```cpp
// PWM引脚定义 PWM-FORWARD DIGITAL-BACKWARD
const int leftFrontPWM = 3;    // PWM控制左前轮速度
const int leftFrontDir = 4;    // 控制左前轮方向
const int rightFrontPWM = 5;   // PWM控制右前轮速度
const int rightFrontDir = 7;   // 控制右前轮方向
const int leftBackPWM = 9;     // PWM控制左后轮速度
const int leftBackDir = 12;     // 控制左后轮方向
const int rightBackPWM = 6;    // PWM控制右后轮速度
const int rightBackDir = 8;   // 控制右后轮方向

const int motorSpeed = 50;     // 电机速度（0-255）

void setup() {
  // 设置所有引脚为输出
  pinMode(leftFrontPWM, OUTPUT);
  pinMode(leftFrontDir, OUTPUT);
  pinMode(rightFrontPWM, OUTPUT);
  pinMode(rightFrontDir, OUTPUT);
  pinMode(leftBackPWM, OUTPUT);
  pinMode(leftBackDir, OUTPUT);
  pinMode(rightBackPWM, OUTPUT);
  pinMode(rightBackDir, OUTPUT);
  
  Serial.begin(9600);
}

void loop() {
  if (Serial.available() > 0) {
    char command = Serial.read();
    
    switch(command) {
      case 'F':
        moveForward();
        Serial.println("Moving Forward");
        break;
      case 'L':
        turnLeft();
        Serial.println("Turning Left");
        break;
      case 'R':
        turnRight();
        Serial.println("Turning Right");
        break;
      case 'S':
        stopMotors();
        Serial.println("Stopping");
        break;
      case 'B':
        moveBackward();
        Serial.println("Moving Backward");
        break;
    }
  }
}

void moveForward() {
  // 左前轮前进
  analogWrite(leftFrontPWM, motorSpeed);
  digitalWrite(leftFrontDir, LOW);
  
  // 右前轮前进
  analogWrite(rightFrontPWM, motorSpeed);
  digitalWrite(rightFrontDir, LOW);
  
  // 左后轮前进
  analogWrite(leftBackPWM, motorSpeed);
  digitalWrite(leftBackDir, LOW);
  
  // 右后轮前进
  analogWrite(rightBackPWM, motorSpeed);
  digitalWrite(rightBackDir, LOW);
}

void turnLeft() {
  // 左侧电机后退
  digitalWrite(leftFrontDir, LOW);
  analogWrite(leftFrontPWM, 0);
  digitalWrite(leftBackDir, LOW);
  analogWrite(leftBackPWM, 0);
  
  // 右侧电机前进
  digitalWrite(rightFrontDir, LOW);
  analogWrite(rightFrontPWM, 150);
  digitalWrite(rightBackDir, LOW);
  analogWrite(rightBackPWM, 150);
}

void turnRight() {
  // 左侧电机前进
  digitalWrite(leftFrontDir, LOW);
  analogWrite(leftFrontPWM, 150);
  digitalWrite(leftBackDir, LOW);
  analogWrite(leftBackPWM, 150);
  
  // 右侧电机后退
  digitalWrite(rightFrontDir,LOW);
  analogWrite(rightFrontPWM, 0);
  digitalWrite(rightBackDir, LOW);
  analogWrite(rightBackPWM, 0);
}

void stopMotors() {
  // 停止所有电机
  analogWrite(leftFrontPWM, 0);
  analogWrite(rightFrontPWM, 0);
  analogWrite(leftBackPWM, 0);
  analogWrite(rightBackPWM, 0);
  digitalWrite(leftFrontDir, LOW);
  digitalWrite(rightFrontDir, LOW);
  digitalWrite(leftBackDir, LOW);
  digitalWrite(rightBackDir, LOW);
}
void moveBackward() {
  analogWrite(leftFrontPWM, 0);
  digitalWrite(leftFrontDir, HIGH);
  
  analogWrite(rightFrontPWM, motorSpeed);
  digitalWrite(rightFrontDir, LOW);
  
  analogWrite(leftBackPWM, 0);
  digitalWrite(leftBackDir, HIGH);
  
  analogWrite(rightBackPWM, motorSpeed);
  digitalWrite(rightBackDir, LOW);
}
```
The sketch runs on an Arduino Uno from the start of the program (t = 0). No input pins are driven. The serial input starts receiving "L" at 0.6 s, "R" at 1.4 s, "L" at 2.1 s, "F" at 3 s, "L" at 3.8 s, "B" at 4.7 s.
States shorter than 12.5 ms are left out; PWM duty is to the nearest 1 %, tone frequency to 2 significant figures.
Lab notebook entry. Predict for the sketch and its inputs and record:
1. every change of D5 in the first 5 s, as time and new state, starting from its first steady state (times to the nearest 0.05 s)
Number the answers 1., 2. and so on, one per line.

1. 0 s low; 0.6 s PWM 59 %; 1.4 s low; 2.1 s PWM 59 %; 3 s PWM 20 %; 3.8 s PWM 59 %; 4.7 s PWM 20 %
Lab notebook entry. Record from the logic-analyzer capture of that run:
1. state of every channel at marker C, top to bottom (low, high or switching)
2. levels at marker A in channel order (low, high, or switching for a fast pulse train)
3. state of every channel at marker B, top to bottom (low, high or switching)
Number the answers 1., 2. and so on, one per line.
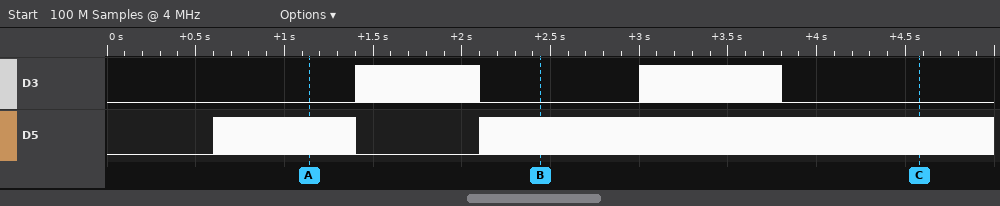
1. D3 low, D5 switching
2. D3 low, D5 switching
3. D3 low, D5 switching
